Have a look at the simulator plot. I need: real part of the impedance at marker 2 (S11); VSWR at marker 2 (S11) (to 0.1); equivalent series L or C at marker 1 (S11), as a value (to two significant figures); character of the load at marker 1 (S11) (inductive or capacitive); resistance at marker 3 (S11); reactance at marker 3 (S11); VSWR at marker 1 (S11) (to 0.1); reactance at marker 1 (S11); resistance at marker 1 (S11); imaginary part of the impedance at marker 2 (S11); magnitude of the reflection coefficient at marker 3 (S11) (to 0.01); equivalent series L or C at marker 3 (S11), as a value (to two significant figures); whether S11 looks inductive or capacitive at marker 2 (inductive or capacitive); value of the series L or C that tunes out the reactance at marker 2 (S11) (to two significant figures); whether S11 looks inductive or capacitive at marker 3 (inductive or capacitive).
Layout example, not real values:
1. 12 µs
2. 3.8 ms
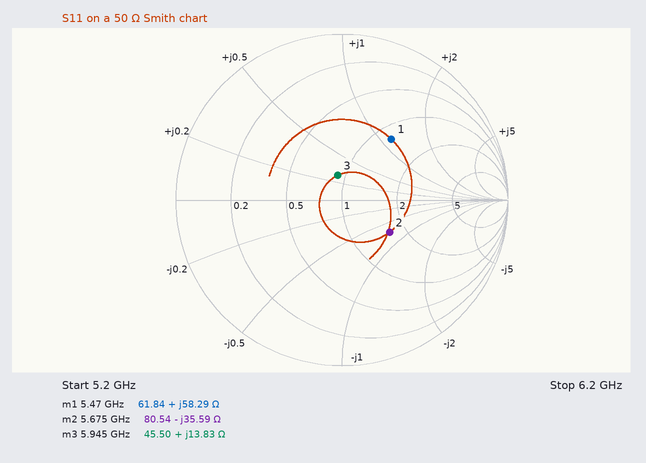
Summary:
1. 80.54 Ω
2. 2.1
3. 1.7 nH
4. inductive
5. 45.50 Ω
6. +13.83 Ω
7. 2.8
8. +58.29 Ω
9. 61.84 Ω
10. -35.59 Ω
11. 0.15
12. 370 pH
13. capacitive
14. 1.00 nH
15. inductive
